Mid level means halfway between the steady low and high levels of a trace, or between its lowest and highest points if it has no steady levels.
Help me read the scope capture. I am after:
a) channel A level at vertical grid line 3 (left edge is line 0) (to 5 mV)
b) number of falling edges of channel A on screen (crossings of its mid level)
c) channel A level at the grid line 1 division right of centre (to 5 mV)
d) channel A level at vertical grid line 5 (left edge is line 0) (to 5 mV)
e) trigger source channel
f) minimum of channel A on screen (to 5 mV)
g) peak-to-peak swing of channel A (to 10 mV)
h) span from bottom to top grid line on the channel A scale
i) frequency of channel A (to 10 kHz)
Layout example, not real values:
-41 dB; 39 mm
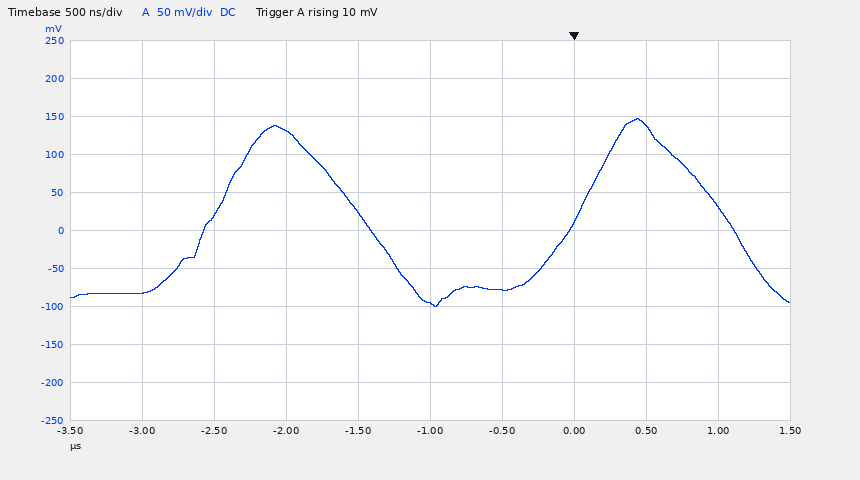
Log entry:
130 mV; 2; -80 mV; -95 mV; channel A; -100 mV; 250 mV; 500 mV; 400 kHz
